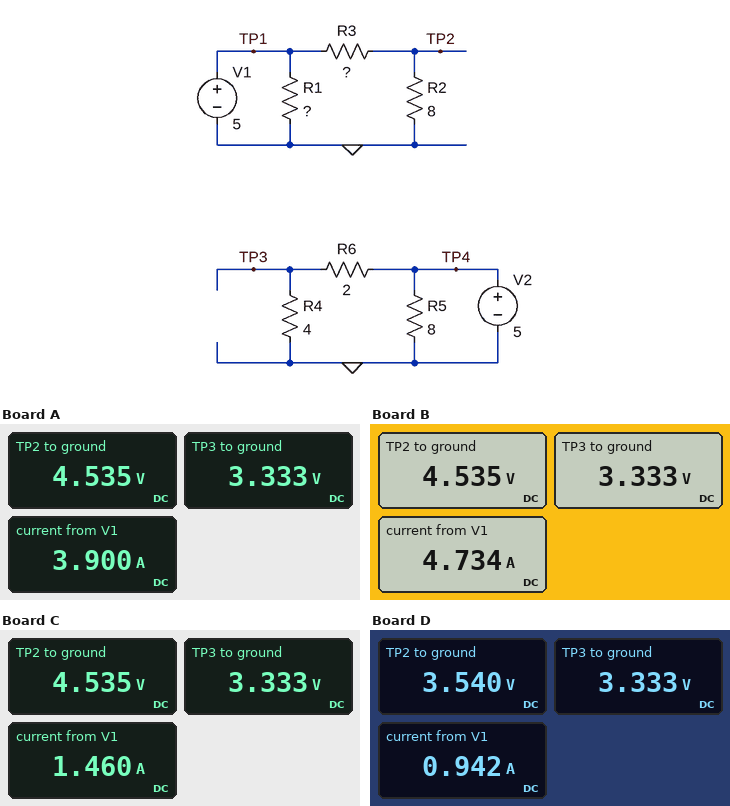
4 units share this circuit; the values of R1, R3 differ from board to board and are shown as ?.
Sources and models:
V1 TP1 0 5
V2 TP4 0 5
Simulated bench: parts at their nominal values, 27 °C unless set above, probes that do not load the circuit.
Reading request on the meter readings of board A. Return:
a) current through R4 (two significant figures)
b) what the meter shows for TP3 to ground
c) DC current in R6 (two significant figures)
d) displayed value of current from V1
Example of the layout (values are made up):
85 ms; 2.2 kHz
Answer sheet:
830 mA; 3.333 V; 830 mA; 3.900 A
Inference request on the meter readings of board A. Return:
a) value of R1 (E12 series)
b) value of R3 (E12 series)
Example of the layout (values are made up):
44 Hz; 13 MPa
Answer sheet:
1.5 Ω; 0.82 Ω
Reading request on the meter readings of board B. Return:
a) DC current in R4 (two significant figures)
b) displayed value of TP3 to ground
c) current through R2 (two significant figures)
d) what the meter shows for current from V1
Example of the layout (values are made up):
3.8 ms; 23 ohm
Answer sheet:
830 mA; 3.333 V; 570 mA; 4.734 A
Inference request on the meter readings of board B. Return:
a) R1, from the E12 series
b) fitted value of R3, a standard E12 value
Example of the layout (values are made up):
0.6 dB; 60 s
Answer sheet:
1.2 Ω; 0.82 Ω
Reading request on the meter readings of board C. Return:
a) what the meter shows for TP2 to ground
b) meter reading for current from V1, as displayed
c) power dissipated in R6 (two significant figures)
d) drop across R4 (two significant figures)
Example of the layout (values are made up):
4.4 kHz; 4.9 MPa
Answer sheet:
4.535 V; 1.460 A; 1.4 W; 3.3 V
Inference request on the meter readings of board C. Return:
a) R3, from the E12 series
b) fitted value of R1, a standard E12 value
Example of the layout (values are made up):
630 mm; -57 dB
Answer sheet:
0.82 Ω; 5.6 Ω
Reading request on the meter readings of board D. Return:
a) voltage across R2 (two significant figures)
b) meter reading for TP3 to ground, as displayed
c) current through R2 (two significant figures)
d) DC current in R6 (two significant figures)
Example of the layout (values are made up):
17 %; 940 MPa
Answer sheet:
3.5 V; 3.333 V; 440 mA; 830 mA
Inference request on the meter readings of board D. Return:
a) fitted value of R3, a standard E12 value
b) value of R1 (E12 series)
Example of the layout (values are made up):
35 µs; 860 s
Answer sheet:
3.3 Ω; 10 Ω
